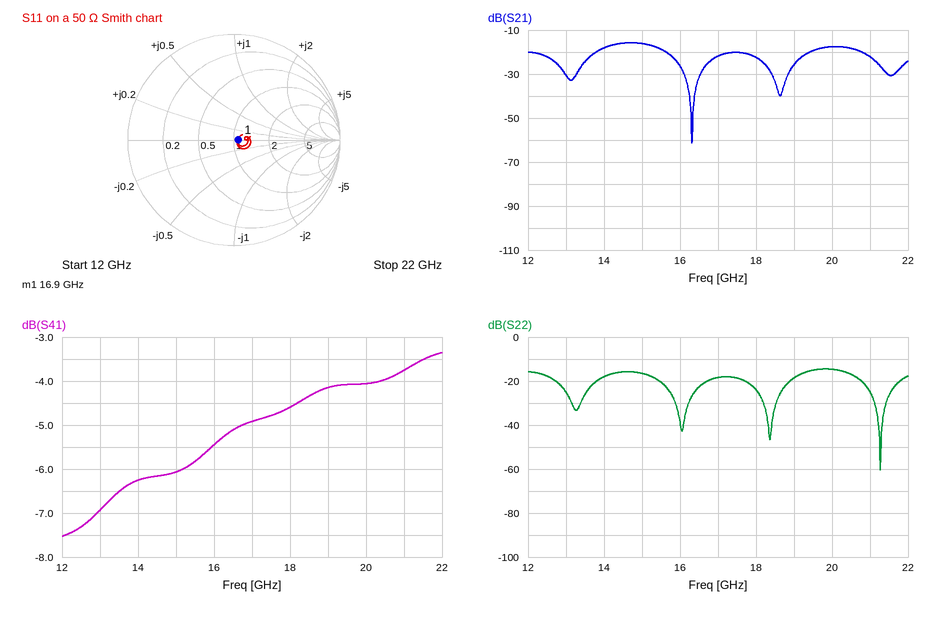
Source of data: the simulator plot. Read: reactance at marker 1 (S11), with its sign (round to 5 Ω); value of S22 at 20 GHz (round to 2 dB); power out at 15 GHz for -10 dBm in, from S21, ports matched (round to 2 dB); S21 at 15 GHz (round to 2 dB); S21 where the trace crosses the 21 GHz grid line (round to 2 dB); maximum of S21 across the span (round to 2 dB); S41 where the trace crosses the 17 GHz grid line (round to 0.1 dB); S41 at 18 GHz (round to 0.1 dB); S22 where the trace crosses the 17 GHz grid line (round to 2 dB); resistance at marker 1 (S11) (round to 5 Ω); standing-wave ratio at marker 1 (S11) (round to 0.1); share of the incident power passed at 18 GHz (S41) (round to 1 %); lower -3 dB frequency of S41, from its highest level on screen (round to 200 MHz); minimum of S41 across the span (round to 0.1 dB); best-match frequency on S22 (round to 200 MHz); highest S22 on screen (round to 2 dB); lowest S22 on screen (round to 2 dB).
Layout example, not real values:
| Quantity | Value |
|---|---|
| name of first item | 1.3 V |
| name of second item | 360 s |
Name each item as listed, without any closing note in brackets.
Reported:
| Quantity | Value |
|---|---|
| reactance at marker 1 (S11), with its sign | 0 Ω |
| value of S22 at 20 GHz | -14 dB |
| power out at 15 GHz for -10 dBm in, from S21, ports matched | -26 dBm |
| S21 at 15 GHz | -16 dB |
| S21 where the trace crosses the 21 GHz grid line | -22 dB |
| maximum of S21 across the span | -16 dB |
| S41 where the trace crosses the 17 GHz grid line | -4.9 dB |
| S41 at 18 GHz | -4.6 dB |
| S22 where the trace crosses the 17 GHz grid line | -18 dB |
| resistance at marker 1 (S11) | 55 Ω |
| standing-wave ratio at marker 1 (S11) | 1.1 |
| share of the incident power passed at 18 GHz (S41) | 35 % |
| lower -3 dB frequency of S41, from its highest level on screen | 13.8 GHz |
| minimum of S41 across the span | -7.5 dB |
| best-match frequency on S22 | 21.2 GHz |
| highest S22 on screen | -14 dB |
| lowest S22 on screen | -60 dB |
